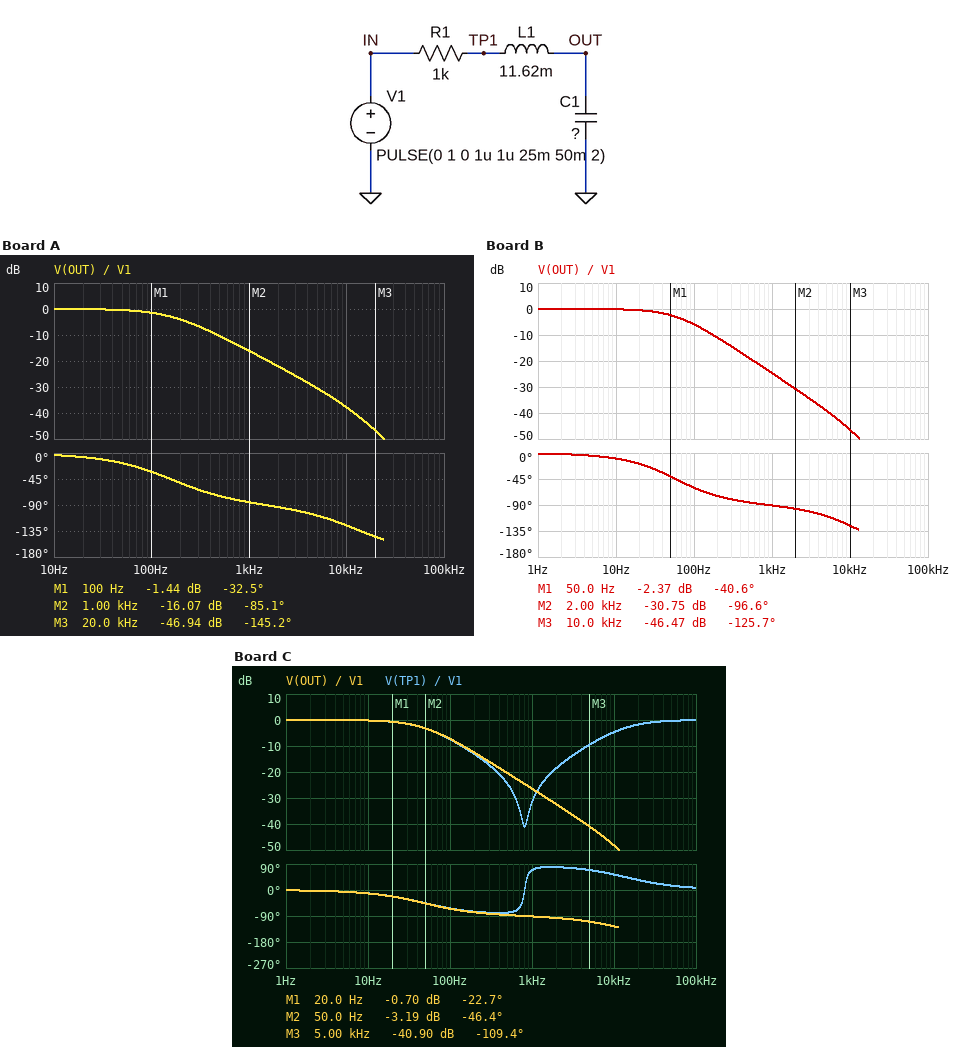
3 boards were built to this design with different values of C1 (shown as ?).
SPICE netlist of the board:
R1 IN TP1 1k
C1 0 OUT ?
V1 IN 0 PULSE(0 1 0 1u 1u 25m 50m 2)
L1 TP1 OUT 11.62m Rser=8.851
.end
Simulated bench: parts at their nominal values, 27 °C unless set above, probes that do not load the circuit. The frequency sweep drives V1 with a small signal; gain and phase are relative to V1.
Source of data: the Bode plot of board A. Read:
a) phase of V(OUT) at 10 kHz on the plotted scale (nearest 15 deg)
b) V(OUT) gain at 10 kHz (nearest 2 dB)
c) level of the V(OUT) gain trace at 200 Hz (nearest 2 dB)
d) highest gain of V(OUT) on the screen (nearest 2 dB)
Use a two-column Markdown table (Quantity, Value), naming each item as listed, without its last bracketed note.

| Quantity | Value |
|---|---|
| phase of V(OUT) at 10 kHz on the plotted scale | -120 deg |
| V(OUT) gain at 10 kHz | -38 dB |
| level of the V(OUT) gain trace at 200 Hz | -4 dB |
| highest gain of V(OUT) on the screen | 0 dB |
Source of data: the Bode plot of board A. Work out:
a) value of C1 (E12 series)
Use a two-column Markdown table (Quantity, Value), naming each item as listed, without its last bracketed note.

| Quantity | Value |
|---|---|
| value of C1 | 1 µF |
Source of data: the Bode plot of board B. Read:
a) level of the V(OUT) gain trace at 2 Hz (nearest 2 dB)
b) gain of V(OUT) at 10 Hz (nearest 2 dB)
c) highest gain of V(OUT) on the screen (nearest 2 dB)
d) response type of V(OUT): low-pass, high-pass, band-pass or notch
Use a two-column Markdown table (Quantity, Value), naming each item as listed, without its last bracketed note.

| Quantity | Value |
|---|---|
| level of the V(OUT) gain trace at 2 Hz | 0 dB |
| gain of V(OUT) at 10 Hz | 0 dB |
| highest gain of V(OUT) on the screen | 0 dB |
| response type of V(OUT): low-pass, high-pass, band-pass or notch | low-pass |
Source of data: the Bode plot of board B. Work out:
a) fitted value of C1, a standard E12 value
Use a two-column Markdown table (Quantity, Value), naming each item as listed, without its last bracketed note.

| Quantity | Value |
|---|---|
| fitted value of C1, a standard E12 value | 2.7 µF |
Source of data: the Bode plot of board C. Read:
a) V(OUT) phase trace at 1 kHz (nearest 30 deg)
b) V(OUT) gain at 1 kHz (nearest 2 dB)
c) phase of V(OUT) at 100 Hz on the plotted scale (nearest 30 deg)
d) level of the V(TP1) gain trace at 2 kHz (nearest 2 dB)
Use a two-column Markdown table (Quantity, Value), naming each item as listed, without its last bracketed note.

| Quantity | Value |
|---|---|
| V(OUT) phase trace at 1 kHz | -90 deg |
| V(OUT) gain at 1 kHz | -26 dB |
| phase of V(OUT) at 100 Hz on the plotted scale | -60 deg |
| level of the V(TP1) gain trace at 2 kHz | -18 dB |
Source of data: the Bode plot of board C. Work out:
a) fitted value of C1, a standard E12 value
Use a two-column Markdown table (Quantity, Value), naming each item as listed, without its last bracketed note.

| Quantity | Value |
|---|---|
| fitted value of C1, a standard E12 value | 3.3 µF |
